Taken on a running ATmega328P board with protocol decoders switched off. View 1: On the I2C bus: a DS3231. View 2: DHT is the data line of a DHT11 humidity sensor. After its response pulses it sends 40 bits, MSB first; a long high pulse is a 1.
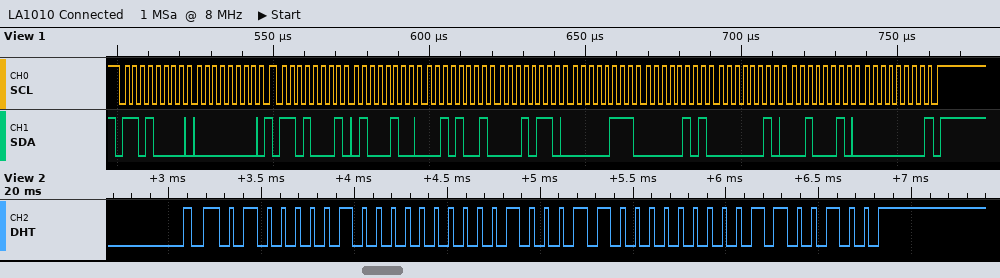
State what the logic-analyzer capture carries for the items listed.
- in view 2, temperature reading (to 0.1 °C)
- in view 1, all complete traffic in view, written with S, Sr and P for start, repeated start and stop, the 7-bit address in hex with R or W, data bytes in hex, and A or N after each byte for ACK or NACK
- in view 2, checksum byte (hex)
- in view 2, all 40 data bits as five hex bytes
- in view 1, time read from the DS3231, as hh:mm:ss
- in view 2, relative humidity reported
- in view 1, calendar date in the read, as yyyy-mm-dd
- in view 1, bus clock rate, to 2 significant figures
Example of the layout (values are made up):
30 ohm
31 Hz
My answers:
35.0 °C
S 68W A 00 A Sr 68R A 44 A 29 A 16 A 07 A 05 A 02 A 22 A 00 N P
0x64
41 00 23 00 64
16:29:44
65 %
2022-02-05
400 kHz
